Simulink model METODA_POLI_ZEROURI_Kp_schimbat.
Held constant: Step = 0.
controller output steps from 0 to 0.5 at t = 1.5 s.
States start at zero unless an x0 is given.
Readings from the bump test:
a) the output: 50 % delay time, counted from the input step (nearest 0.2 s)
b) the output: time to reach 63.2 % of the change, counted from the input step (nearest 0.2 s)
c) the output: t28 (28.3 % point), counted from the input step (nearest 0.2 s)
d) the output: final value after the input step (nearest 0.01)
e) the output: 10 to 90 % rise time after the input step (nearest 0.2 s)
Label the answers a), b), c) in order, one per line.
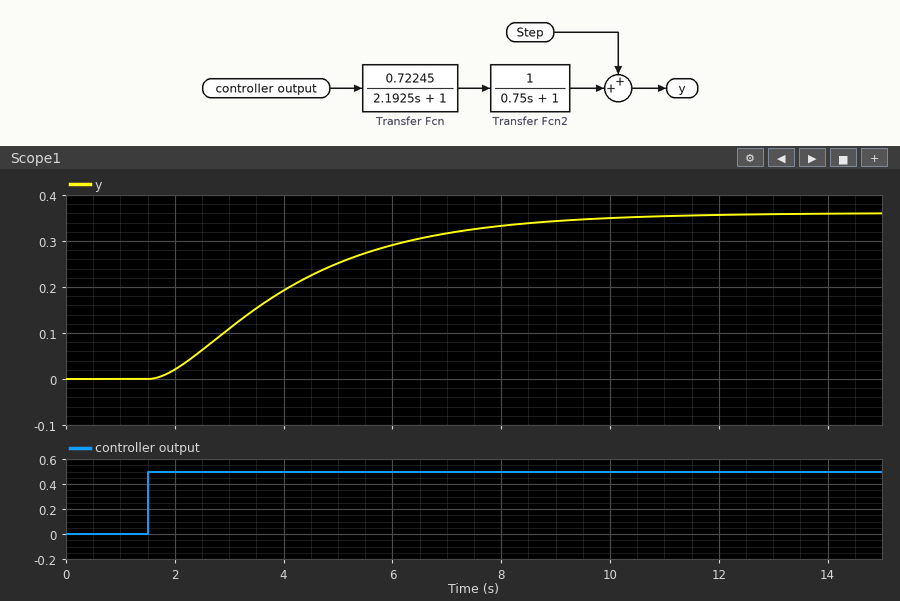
a) 2.4 s
b) 3.0 s
c) 1.4 s
d) 0.36
e) 5.2 s
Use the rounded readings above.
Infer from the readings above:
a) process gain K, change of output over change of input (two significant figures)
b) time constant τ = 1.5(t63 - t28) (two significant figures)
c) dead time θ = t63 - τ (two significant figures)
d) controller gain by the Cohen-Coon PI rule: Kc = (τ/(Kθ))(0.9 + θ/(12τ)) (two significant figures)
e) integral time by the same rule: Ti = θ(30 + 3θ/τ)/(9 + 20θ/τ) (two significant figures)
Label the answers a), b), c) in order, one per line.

a) 0.72
b) 2.4 s
c) 0.60 s
d) 5.1
e) 1.3 s
